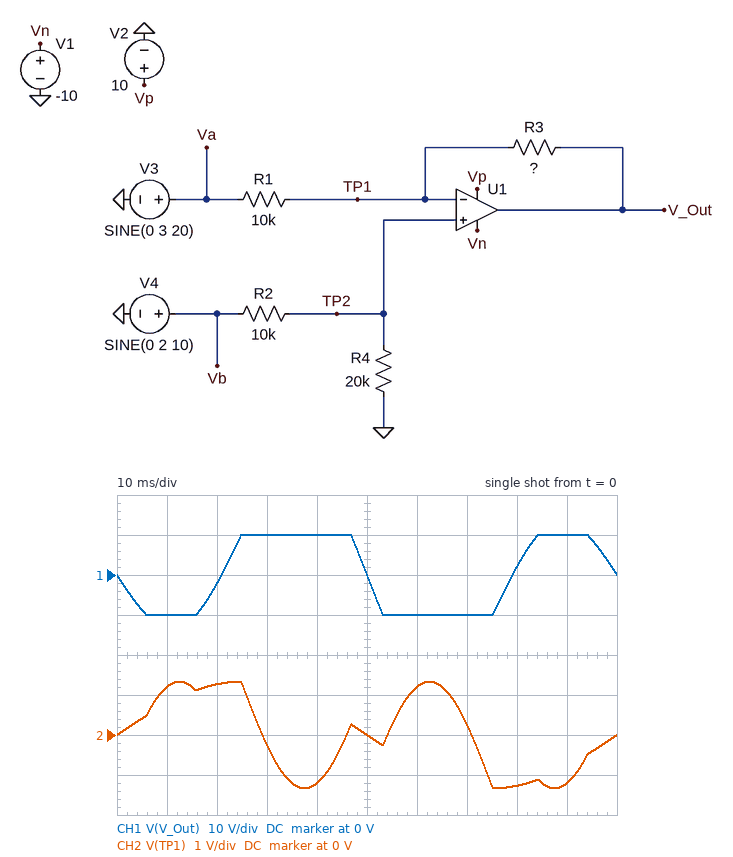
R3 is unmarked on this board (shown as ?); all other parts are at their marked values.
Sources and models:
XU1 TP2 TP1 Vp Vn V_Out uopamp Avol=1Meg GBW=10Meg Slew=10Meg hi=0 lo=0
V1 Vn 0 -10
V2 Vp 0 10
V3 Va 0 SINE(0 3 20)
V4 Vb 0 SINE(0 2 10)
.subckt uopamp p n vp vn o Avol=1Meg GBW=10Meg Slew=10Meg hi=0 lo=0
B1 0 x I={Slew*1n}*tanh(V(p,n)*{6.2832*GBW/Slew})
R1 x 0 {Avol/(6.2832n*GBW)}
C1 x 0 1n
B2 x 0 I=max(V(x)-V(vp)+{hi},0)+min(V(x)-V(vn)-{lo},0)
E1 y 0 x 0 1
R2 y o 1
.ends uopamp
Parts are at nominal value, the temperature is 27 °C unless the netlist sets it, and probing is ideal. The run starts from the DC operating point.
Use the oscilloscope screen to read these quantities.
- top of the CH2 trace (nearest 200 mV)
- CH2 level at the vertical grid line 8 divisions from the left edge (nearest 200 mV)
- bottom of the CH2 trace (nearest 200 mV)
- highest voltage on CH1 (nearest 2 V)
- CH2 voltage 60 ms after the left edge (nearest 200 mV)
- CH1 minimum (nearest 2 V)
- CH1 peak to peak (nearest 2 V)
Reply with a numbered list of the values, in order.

1. 1.4 V
2. -1.2 V
3. -1.4 V
4. 10 V
5. 1.2 V
6. -10 V
7. 20 V
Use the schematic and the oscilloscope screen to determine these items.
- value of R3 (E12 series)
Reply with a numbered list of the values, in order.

1. 68 kΩ
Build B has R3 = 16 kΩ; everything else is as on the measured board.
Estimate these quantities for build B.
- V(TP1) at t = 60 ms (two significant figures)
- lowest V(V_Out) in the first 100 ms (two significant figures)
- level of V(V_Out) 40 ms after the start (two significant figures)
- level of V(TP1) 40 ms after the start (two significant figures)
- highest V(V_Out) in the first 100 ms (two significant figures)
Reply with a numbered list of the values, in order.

1. -780 mV
2. -7.4 V
3. 6.6 V
4. 780 mV
5. 7.4 V
